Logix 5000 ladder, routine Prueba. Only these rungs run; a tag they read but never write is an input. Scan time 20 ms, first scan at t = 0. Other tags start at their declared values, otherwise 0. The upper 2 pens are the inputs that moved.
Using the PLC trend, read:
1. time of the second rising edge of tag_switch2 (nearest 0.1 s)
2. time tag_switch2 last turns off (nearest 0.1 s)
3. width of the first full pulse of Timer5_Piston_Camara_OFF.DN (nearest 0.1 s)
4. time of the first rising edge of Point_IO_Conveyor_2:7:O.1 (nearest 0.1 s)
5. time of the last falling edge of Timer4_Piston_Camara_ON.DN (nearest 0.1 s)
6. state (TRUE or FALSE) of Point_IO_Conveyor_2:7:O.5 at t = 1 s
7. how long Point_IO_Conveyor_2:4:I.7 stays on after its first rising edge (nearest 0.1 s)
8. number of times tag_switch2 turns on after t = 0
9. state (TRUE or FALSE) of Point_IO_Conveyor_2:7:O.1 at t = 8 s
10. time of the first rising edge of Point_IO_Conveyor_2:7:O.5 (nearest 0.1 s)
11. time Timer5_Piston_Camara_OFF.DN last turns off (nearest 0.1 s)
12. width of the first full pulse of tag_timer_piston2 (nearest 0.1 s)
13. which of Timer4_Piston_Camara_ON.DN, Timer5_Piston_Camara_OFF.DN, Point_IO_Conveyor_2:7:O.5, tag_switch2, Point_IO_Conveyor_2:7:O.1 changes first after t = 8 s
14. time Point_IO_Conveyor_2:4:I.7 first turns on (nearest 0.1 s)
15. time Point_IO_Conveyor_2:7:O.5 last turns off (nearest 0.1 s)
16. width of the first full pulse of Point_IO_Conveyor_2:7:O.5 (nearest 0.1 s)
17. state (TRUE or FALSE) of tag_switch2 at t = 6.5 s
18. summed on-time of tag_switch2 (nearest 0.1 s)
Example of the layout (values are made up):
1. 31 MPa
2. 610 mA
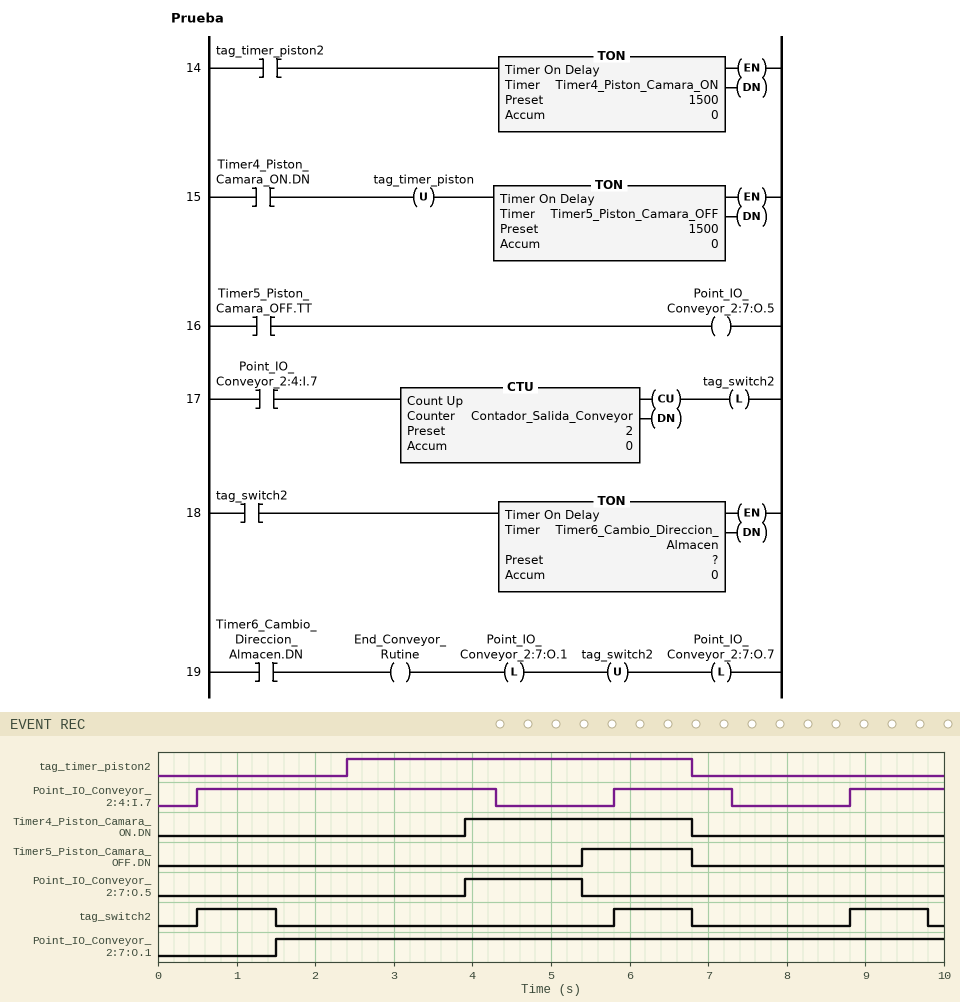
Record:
1. 5.8 s
2. 9.8 s
3. 1.4 s
4. 1.5 s
5. 6.8 s
6. FALSE
7. 3.8 s
8. 3
9. TRUE
10. 3.9 s
11. 6.8 s
12. 4.4 s
13. tag_switch2
14. 0.5 s
15. 5.4 s
16. 1.5 s
17. TRUE
18. 3.0 s
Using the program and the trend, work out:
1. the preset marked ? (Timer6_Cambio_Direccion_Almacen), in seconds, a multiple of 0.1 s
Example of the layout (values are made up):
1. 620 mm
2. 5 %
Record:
1. 1.0 s
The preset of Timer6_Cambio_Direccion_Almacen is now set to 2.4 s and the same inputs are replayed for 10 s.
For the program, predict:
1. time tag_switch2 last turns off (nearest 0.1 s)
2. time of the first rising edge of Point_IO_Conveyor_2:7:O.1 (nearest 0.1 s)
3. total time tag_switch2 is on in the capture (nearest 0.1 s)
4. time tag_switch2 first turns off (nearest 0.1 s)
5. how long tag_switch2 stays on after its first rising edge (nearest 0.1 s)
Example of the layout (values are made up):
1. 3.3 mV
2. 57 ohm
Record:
1. 8.2 s
2. 2.9 s
3. 6.0 s
4. 2.9 s
5. 2.4 s
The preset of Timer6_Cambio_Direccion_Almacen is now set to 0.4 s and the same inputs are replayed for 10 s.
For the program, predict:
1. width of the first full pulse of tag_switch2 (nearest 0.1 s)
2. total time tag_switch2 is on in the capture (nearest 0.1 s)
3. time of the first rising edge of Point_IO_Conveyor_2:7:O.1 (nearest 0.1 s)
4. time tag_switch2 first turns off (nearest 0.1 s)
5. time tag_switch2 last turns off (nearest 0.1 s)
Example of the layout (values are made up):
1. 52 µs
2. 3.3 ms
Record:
1. 0.4 s
2. 1.2 s
3. 0.9 s
4. 0.9 s
5. 9.2 s
